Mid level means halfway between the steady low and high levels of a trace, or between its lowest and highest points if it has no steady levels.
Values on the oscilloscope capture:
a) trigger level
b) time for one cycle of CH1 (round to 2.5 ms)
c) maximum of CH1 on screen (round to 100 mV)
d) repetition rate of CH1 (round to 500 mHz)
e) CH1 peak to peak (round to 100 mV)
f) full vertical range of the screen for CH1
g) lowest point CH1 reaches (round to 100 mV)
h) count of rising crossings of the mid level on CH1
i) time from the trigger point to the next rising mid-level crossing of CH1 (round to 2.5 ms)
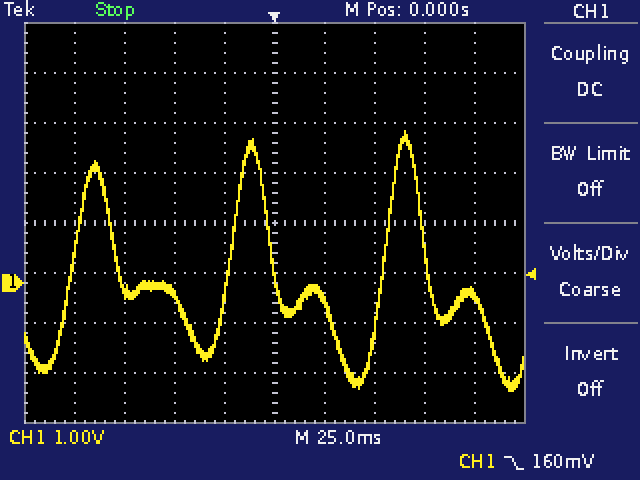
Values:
160 mV
77.5 ms
3.0 V
13.0 Hz
5.2 V
8 V
-2.2 V
3
55.0 ms
